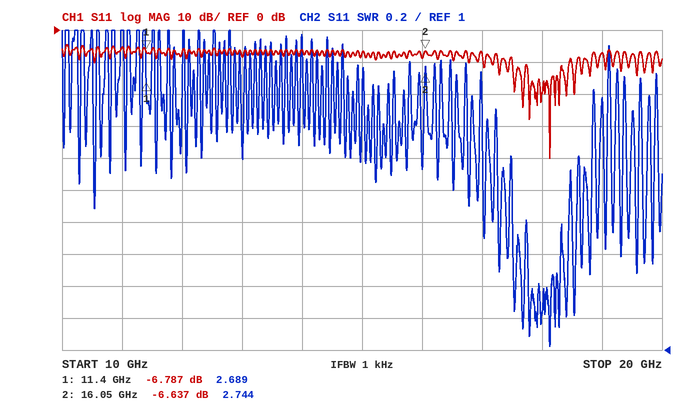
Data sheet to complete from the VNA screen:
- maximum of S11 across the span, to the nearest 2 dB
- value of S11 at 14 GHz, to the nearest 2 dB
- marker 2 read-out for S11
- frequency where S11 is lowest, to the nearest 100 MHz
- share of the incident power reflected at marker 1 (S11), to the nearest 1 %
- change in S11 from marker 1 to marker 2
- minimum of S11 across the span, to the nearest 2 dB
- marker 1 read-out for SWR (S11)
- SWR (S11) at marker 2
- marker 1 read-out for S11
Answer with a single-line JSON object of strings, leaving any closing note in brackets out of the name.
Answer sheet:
{"maximum of S11 across the span, to the nearest 2 dB": "-4 dB", "value of S11 at 14 GHz, to the nearest 2 dB": "-6 dB", "marker 2 read-out for S11": "-6.637 dB", "frequency where S11 is lowest, to the nearest 100 MHz": "18.1 GHz", "share of the incident power reflected at marker 1 (S11), to the nearest 1 %": "21 %", "change in S11 from marker 1 to marker 2": "0.150 dB", "minimum of S11 across the span, to the nearest 2 dB": "-40 dB", "marker 1 read-out for SWR": "2.689", "SWR (S11) at marker 2": "2.744", "marker 1 read-out for S11": "-6.787 dB"}
